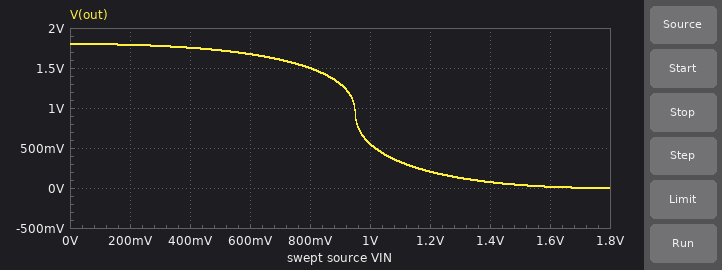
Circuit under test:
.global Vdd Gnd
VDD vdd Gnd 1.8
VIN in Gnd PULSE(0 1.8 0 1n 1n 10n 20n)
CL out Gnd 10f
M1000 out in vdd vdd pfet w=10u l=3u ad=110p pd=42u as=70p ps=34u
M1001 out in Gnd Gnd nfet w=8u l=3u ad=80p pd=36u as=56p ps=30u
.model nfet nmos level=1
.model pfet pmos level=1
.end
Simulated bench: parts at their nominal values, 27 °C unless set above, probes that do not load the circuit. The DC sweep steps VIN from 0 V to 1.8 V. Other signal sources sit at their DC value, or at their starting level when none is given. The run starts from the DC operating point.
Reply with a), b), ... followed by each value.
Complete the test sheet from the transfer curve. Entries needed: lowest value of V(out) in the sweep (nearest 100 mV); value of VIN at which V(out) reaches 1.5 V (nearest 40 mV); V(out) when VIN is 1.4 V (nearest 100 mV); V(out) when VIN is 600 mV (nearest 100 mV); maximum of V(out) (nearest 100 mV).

a) 0 V
b) 800 mV
c) 100 mV
d) 1.7 V
e) 1.8 V
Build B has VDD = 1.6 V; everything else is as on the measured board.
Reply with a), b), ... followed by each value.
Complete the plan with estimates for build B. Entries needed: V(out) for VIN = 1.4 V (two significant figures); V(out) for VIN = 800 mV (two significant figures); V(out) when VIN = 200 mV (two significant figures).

a) 18 mV
b) 1.2 V
c) 1.6 V
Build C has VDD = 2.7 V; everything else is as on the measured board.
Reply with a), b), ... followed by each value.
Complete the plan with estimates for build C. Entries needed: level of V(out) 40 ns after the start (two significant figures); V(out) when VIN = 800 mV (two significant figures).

a) 2.7 V
b) 2.6 V
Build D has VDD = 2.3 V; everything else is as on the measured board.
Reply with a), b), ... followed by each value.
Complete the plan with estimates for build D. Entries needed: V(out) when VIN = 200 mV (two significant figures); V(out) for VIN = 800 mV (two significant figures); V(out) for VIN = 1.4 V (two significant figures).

a) 2.3 V
b) 2.1 V
c) 430 mV
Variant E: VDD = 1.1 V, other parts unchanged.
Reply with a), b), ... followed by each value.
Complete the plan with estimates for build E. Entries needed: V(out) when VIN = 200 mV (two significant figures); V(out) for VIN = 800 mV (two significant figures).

a) 1.1 V
b) 74 mV
